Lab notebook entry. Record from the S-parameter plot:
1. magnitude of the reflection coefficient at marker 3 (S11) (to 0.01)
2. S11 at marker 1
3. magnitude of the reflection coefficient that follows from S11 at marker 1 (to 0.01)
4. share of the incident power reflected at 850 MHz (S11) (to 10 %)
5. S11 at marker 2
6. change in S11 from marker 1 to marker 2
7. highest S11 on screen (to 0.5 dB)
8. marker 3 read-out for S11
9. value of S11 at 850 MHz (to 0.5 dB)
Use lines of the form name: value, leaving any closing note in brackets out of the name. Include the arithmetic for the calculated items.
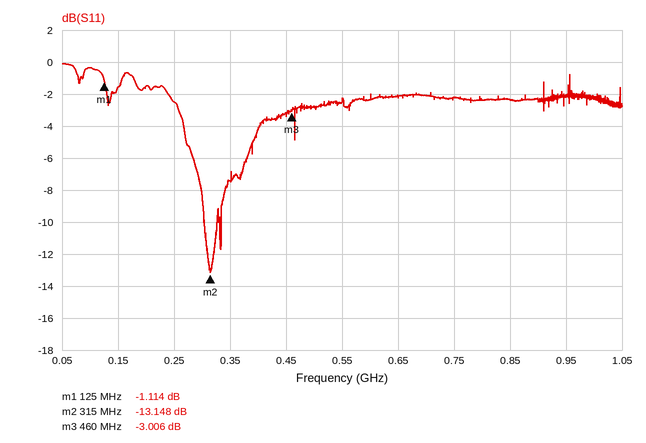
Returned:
magnitude of the reflection coefficient at marker 3 (S11): 10^(-3.006/20) ≈ 0.71
S11 at marker 1: -1.114 dB
magnitude of the reflection coefficient that follows from S11 at marker 1: 10^(-1.114/20) ≈ 0.88
share of the incident power reflected at 850 MHz (S11): 10^(-2.5/10) ≈ 56.2 %, so 60 % to the nearest 10 %
S11 at marker 2: -13.148 dB
change in S11 from marker 1 to marker 2: -13.148 − (-1.114) = -12.034 dB
highest S11 on screen: 0.0 dB
marker 3 read-out for S11: -3.006 dB
value of S11 at 850 MHz: -2.5 dB
